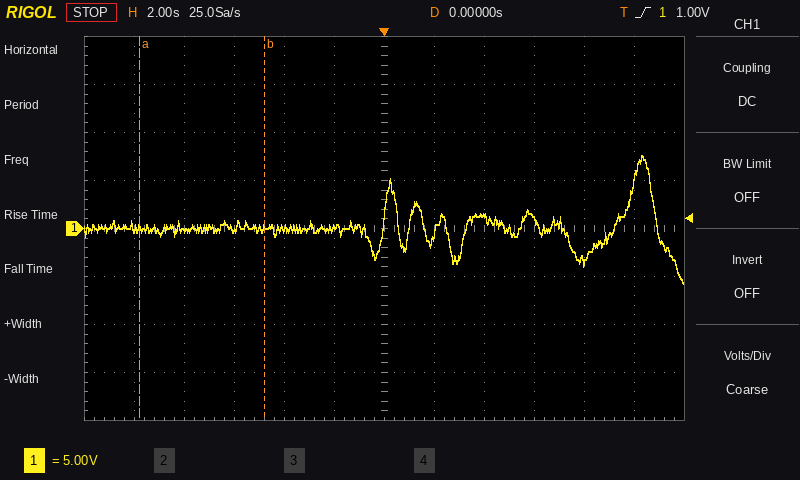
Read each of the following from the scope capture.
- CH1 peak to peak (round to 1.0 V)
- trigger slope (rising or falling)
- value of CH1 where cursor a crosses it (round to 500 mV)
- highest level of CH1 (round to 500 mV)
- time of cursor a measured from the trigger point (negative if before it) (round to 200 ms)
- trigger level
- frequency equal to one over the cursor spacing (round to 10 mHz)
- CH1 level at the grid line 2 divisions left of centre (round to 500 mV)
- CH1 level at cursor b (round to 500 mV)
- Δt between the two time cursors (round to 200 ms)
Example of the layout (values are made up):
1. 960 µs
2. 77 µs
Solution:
1. 13.0 V
2. rising
3. 0.0 V
4. 7.5 V
5. -9.8 s
6. 1.00 V
7. 200 mHz
8. 0.0 V
9. 0.0 V
10. 5.0 s
